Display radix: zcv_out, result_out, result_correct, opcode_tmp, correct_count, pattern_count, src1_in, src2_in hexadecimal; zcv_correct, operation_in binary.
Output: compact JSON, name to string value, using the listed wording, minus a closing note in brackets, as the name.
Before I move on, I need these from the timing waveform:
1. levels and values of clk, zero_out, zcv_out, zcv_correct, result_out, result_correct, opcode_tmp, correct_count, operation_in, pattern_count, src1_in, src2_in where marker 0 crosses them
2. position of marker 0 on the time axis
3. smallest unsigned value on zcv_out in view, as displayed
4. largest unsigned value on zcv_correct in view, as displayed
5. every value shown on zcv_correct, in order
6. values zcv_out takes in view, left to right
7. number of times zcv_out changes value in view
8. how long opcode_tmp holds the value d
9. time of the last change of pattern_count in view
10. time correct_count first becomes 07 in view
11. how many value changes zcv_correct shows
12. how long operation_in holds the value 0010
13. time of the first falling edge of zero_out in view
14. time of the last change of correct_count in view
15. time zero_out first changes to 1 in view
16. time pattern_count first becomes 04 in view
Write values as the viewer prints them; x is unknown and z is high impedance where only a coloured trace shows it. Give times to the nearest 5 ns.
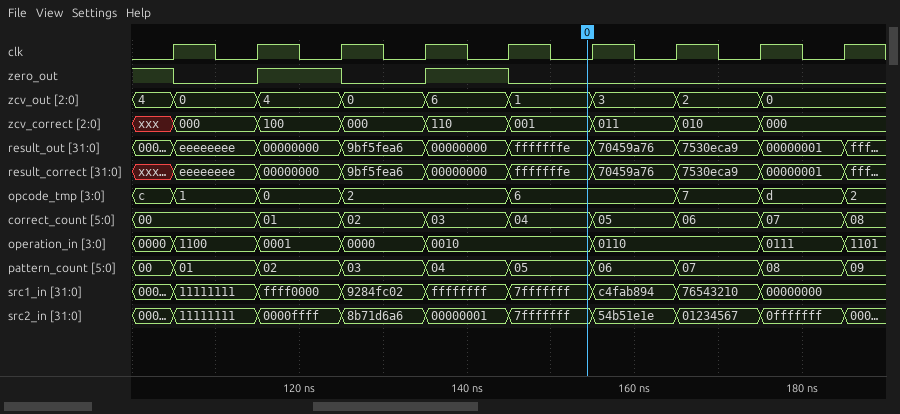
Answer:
{"levels and values of clk, zero_out, zcv_out, zcv_correct, result_out, result_correct, opcode_tmp, correct_count, operation_in, pattern_count, src1_in, src2_in where marker 0 crosses them": "clk=0, zero_out=0, zcv_out=1, zcv_correct=001, result_out=fffffffe, result_correct=fffffffe, opcode_tmp=6, correct_count=04, operation_in=0010, pattern_count=05, src1_in=7fffffff, src2_in=7fffffff", "position of marker 0 on the time axis": "155 ns", "smallest unsigned value on zcv_out in view, as displayed": "0", "largest unsigned value on zcv_correct in view, as displayed": "110", "every value shown on zcv_correct, in order": "xxx, 000, 100, 000, 110, 001, 011, 010, 000", "values zcv_out takes in view, left to right": "4, 0, 4, 0, 6, 1, 3, 2, 0", "number of times zcv_out changes value in view": "8", "how long opcode_tmp holds the value d": "10 ns", "time of the last change of pattern_count in view": "185 ns", "time correct_count first becomes 07 in view": "175 ns", "how many value changes zcv_correct shows": "8", "how long operation_in holds the value 0010": "20 ns", "time of the first falling edge of zero_out in view": "105 ns", "time of the last change of correct_count in view": "185 ns", "time zero_out first changes to 1 in view": "115 ns", "time pattern_count first becomes 04 in view": "135 ns"}
